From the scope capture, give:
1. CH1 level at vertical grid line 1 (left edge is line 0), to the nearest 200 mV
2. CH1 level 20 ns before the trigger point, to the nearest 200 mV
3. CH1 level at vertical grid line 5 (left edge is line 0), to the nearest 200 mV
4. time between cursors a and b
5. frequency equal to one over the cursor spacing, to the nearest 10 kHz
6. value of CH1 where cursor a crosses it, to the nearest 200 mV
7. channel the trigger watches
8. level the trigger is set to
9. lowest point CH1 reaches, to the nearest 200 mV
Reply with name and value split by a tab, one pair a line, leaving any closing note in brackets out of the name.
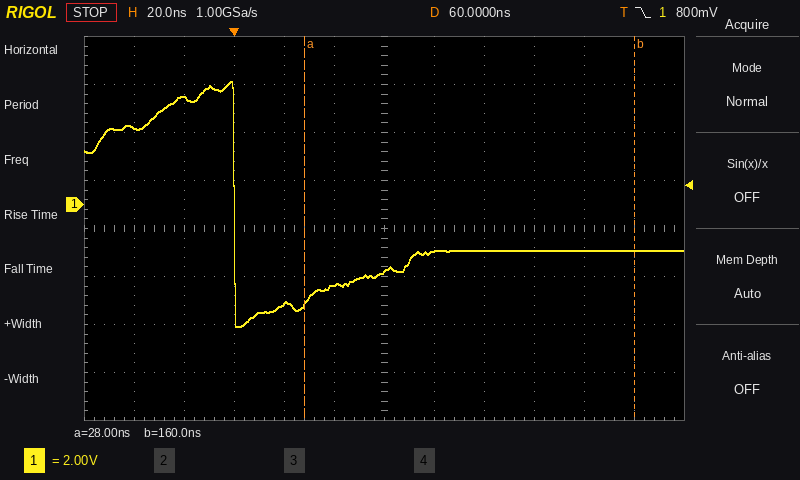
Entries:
CH1 level at vertical grid line 1 (left edge is line 0), to the nearest 200 mV	3.2 V
CH1 level 20 ns before the trigger point, to the nearest 200 mV	4.4 V
CH1 level at vertical grid line 5 (left edge is line 0), to the nearest 200 mV	-3.4 V
time between cursors a and b	132 ns
frequency equal to one over the cursor spacing, to the nearest 10 kHz	7.58 MHz
value of CH1 where cursor a crosses it, to the nearest 200 mV	-4.2 V
channel the trigger watches	CH1
level the trigger is set to	800 mV
lowest point CH1 reaches, to the nearest 200 mV	-5.0 V
